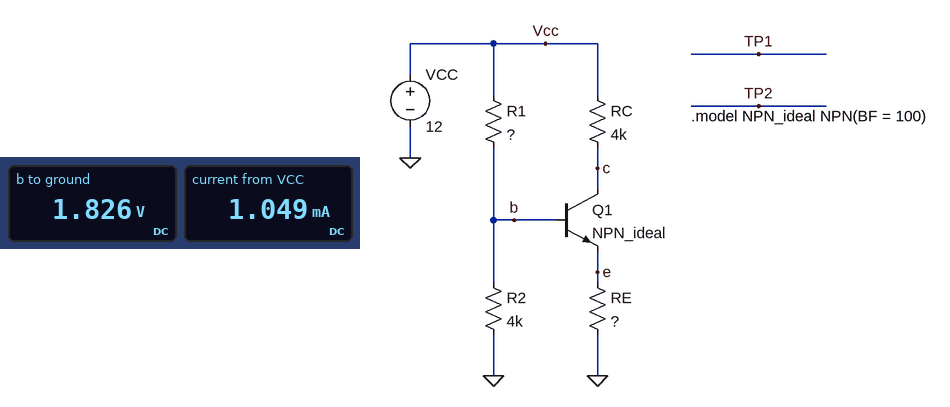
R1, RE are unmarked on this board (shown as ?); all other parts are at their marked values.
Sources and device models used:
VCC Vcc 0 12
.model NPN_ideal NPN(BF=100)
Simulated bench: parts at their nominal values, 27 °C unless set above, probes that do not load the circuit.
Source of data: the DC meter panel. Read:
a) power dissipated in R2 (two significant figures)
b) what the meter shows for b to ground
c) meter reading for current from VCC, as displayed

830 µW
1.826 V
1.049 mA
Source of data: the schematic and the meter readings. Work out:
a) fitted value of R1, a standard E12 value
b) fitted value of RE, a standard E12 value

22 kΩ
1.8 kΩ
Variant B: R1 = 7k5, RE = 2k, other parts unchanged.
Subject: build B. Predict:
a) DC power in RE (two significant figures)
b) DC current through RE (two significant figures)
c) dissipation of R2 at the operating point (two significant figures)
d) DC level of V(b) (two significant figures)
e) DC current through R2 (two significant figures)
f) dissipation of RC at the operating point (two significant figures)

5.6 mW
1.7 mA
4.3 mW
4.1 V
1.0 mA
11 mW
